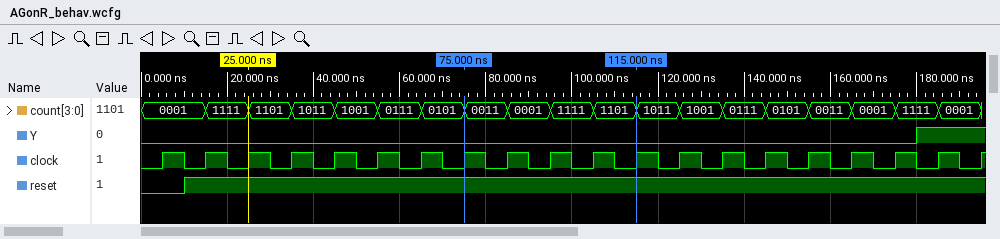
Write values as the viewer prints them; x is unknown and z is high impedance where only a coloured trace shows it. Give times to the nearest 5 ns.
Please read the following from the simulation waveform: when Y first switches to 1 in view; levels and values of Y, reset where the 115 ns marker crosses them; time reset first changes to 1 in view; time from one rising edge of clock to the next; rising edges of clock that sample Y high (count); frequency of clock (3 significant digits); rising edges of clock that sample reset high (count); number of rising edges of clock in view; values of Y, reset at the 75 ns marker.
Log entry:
180 ns
Y=0, reset=1
10 ns
10 ns
2
100 MHz
19
20
Y=0, reset=1
